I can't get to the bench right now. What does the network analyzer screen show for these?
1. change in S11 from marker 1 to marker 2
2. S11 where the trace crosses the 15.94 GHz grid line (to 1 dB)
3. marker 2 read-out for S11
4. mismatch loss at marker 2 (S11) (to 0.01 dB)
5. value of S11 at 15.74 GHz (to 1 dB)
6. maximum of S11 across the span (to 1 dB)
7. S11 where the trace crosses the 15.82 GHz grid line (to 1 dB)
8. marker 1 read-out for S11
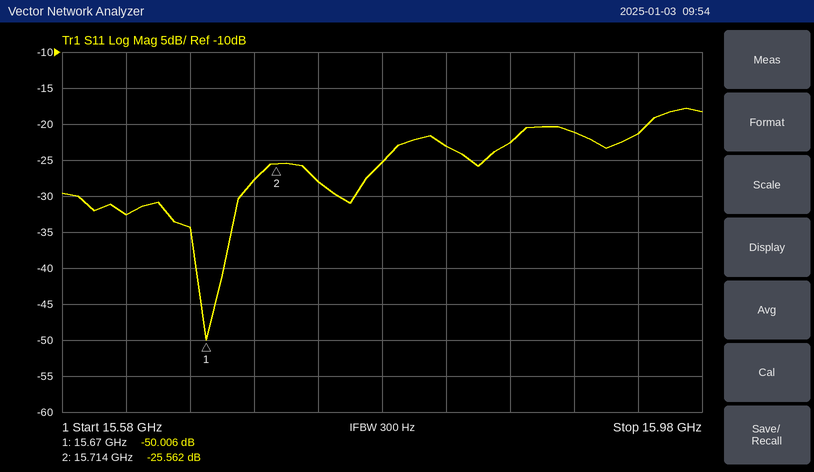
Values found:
24.444 dB
-21 dB
-25.562 dB
0.01 dB
-28 dB
-18 dB
-23 dB
-50.006 dB
